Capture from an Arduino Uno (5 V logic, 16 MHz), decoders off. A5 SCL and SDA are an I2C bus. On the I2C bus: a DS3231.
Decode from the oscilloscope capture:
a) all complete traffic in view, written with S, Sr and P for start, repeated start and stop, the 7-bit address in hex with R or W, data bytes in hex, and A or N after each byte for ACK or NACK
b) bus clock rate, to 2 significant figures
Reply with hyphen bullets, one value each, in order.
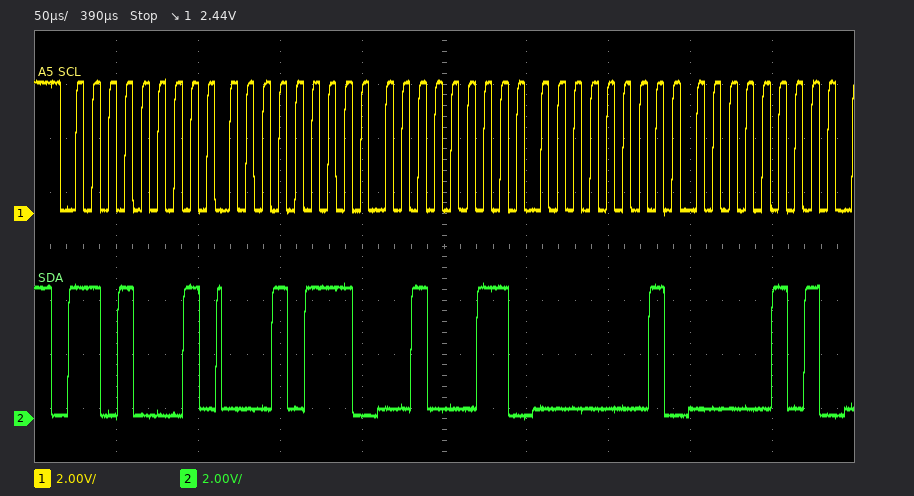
- S 68R A 17 A 23 A 01 A 05 A
- 100 kHz
